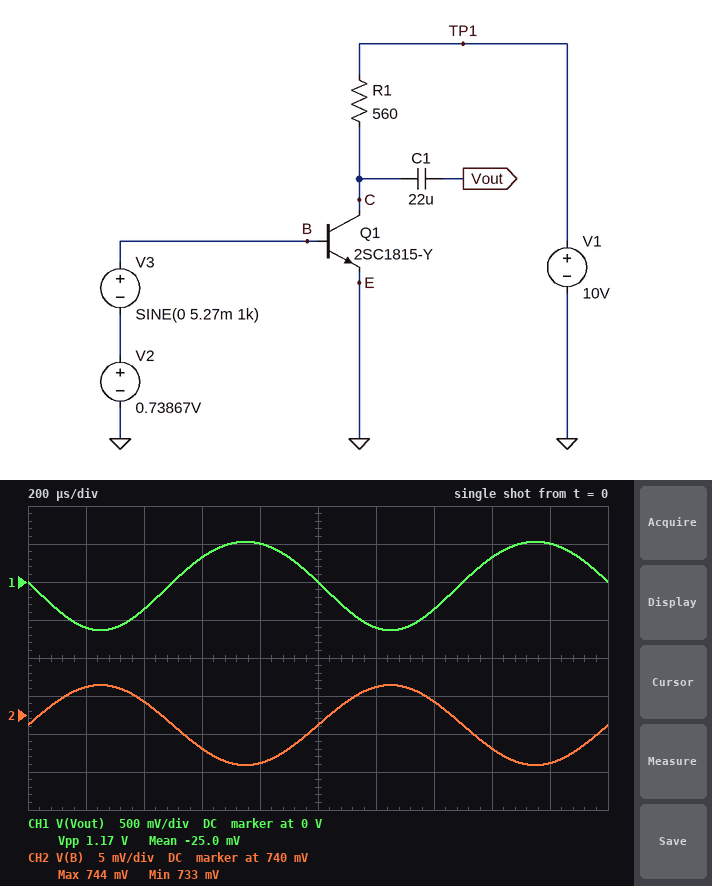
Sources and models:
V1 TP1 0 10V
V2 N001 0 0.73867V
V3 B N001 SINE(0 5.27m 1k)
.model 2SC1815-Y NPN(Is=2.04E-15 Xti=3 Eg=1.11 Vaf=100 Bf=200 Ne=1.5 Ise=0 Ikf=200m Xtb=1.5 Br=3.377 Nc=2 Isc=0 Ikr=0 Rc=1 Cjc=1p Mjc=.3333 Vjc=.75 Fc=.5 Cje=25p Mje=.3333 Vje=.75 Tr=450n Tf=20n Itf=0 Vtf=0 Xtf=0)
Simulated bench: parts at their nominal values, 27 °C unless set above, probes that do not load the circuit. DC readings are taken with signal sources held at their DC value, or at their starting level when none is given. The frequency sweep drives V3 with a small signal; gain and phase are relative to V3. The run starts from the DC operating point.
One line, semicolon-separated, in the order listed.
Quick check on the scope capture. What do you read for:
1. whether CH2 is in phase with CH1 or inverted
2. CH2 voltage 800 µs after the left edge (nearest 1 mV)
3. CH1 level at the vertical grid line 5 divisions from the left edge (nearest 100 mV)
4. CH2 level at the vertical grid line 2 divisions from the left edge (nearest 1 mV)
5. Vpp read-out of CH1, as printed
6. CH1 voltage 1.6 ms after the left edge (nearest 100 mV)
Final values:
inverted; 734 mV; 0 V; 742 mV; 1.17 V; 300 mV
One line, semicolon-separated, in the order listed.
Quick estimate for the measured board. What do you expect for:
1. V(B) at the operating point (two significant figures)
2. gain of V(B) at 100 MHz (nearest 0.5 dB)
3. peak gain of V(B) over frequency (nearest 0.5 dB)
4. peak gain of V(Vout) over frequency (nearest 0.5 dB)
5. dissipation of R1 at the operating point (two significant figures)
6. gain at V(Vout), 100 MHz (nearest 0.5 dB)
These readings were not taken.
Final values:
740 mV; 0 dB; 0 dB; 41.0 dB; 16 mW; 40.5 dB
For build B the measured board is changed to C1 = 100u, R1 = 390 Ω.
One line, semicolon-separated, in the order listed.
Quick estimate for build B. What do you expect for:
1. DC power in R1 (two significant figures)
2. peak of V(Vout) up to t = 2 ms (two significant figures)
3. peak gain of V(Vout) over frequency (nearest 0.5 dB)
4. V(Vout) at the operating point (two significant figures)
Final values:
11 mW; 370 mV; 38.0 dB; 7.9 V
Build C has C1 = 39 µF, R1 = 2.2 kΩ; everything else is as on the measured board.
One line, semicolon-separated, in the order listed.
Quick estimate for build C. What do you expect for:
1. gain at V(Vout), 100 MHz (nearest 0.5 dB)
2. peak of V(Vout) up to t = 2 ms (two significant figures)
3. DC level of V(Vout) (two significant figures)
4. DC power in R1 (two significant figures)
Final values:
0 dB; 840 mV; 72 mV; 45 mW
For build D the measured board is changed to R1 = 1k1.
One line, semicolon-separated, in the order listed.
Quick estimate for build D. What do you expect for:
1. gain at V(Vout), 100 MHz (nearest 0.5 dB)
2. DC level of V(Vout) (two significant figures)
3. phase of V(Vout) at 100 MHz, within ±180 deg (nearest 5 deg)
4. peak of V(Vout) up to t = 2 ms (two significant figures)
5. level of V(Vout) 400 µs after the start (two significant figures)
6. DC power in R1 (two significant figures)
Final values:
45.5 dB; 4.3 V; 160 deg; 990 mV; -670 mV; 30 mW
